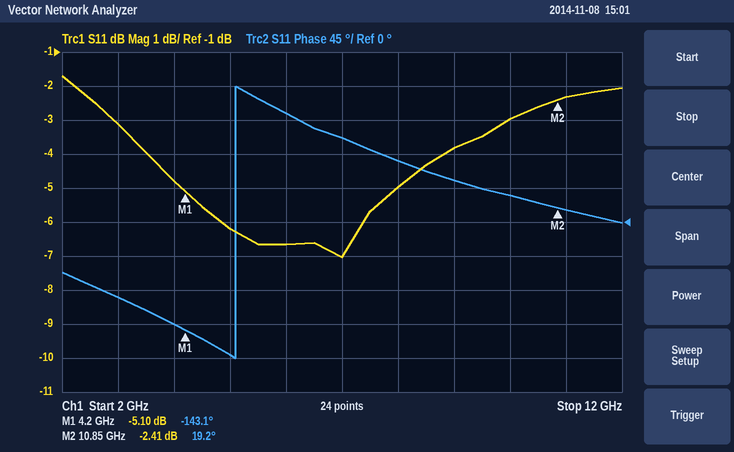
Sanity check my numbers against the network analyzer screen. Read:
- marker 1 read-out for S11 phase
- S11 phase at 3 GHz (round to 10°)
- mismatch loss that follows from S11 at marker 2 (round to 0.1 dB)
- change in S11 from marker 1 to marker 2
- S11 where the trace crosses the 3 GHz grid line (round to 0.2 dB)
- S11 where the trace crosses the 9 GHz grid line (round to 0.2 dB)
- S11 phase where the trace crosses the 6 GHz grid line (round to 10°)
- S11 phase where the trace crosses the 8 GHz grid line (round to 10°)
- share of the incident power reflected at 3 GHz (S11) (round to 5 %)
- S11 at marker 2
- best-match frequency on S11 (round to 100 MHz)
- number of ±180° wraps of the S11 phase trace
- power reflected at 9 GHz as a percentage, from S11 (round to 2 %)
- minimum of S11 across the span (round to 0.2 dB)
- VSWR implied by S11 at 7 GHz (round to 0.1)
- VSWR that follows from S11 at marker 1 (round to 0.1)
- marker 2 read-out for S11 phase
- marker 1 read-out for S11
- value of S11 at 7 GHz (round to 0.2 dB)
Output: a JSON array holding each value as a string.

["-143.1°", "-100°", "3.7 dB", "2.69 dB", "-3.2 dB", "-3.8 dB", "140°", "80°", "50 %", "-2.41 dB", "7.0 GHz", "1", "42 %", "-7.0 dB", "2.6", "3.5", "19.2°", "-5.10 dB", "-7.0 dB"]
